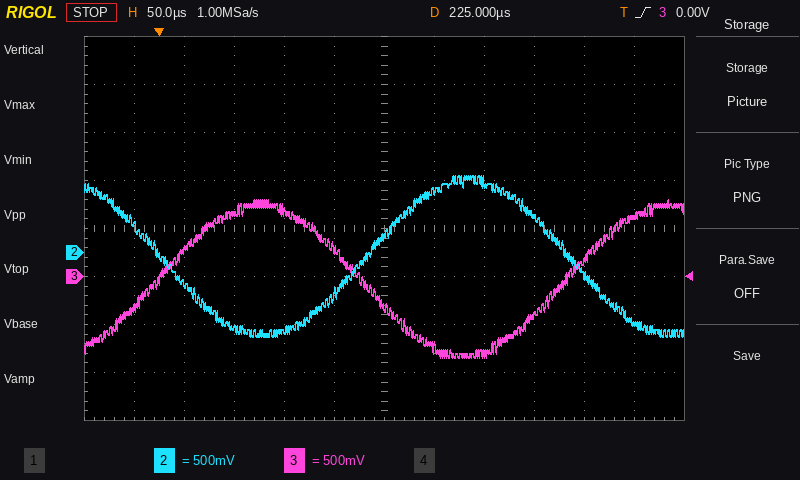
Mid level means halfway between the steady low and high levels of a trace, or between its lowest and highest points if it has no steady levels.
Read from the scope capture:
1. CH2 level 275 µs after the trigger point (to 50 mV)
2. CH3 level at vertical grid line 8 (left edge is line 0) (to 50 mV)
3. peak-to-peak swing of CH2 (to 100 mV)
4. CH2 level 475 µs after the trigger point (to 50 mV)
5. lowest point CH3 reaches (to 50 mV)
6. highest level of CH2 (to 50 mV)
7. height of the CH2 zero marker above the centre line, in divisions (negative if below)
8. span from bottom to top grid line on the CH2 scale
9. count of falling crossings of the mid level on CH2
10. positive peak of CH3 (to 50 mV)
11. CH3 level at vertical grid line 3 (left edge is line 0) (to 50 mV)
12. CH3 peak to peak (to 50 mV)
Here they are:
650 mV
-800 mV
1.70 V
-700 mV
-850 mV
800 mV
-0.5 div
4 V
2
800 mV
650 mV
1.65 V
